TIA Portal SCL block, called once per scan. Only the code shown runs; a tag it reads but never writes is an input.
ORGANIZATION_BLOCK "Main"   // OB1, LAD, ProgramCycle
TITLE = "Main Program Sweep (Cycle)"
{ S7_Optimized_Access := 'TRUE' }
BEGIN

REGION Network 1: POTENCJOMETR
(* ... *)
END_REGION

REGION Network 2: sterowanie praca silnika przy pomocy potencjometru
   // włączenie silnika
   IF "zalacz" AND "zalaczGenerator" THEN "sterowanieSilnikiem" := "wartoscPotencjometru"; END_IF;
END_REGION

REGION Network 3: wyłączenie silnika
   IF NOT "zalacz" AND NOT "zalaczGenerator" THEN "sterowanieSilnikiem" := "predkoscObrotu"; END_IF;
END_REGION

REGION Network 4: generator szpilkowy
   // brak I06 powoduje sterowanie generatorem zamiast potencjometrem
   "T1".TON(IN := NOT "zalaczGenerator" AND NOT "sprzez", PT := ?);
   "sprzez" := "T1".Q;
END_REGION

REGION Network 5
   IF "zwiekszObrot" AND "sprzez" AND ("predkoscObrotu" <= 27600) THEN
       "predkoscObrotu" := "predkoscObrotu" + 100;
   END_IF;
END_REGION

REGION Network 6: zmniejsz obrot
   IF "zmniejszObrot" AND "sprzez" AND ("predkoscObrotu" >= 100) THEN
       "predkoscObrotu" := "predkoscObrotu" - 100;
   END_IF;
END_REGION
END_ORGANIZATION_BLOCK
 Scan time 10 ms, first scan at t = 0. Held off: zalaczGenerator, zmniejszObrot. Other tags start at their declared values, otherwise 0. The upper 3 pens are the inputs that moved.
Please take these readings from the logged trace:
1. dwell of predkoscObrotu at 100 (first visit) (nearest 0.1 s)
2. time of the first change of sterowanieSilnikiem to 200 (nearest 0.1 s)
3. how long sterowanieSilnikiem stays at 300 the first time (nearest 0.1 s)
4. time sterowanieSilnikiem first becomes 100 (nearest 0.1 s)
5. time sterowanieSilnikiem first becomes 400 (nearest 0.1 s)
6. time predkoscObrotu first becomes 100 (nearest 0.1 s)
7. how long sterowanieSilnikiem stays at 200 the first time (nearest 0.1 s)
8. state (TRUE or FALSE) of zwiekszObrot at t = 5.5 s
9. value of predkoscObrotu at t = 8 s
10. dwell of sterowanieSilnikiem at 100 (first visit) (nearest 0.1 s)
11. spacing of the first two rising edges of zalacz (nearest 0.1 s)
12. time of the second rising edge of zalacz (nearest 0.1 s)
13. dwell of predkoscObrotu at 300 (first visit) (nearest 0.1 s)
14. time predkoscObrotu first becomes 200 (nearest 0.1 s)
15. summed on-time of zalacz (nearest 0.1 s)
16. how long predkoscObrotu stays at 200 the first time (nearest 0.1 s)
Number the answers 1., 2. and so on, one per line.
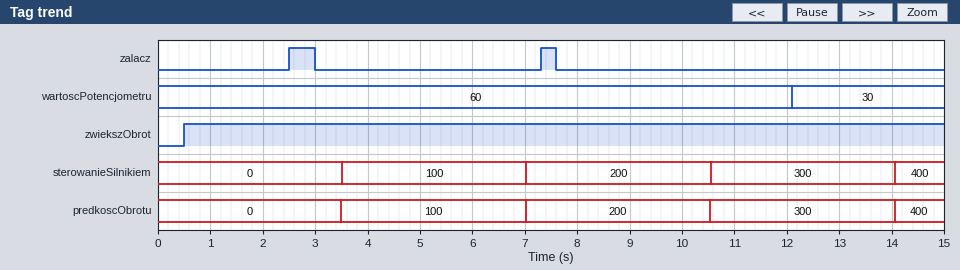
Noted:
1. 3.5 s
2. 7.0 s
3. 3.5 s
4. 3.5 s
5. 14.1 s
6. 3.5 s
7. 3.5 s
8. TRUE
9. 200
10. 3.5 s
11. 4.8 s
12. 7.3 s
13. 3.5 s
14. 7.0 s
15. 0.8 s
16. 3.5 s
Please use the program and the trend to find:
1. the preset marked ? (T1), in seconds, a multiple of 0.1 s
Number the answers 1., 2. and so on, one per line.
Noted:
1. 3.5 s
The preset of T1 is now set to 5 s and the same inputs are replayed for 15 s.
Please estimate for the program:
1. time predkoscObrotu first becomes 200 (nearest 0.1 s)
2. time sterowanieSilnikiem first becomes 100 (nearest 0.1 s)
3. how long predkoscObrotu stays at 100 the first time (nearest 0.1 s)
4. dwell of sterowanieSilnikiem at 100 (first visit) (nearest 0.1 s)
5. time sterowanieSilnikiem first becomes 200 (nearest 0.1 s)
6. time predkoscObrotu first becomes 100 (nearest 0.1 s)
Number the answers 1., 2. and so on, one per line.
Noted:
1. 10.0 s
2. 5.0 s
3. 5.0 s
4. 5.0 s
5. 10.0 s
6. 5.0 s
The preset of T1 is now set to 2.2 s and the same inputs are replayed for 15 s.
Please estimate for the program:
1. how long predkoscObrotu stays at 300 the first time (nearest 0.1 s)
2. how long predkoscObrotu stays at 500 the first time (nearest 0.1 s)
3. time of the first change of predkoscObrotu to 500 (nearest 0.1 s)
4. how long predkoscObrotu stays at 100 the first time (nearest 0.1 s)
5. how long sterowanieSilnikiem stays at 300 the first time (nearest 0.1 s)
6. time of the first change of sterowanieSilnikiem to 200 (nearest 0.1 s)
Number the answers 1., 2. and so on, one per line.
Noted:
1. 2.2 s
2. 2.2 s
3. 11.1 s
4. 2.2 s
5. 2.2 s
6. 4.4 s
